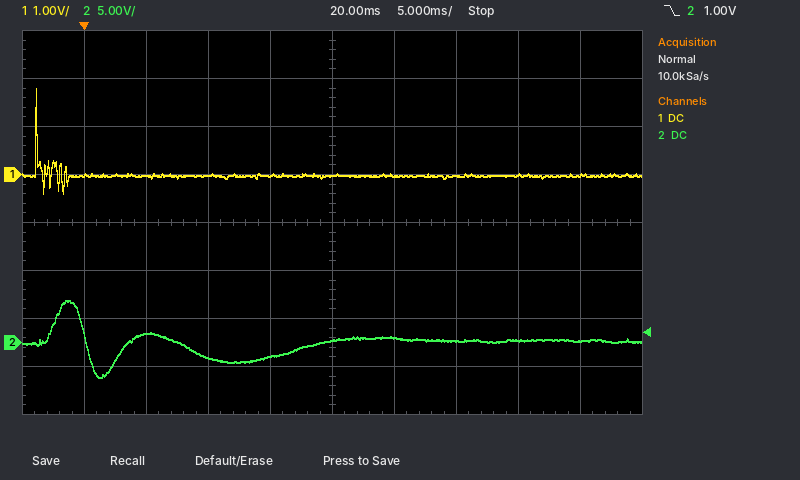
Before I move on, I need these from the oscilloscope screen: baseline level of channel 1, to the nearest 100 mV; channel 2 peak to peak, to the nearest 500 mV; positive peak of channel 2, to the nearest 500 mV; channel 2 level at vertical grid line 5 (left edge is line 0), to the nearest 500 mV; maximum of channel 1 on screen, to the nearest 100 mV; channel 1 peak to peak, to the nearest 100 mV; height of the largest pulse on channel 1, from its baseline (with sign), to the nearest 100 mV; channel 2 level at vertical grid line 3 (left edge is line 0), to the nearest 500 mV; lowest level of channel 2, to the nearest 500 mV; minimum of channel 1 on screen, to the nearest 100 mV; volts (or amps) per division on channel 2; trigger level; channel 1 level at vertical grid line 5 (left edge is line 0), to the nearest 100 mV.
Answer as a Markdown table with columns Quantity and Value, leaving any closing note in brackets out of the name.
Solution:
| Quantity | Value |
|---|---|
| baseline level of channel 1, to the nearest 100 mV | 0.0 V |
| channel 2 peak to peak, to the nearest 500 mV | 8.0 V |
| positive peak of channel 2, to the nearest 500 mV | 4.5 V |
| channel 2 level at vertical grid line 5 (left edge is line 0), to the nearest 500 mV | 0.0 V |
| maximum of channel 1 on screen, to the nearest 100 mV | 1.8 V |
| channel 1 peak to peak, to the nearest 100 mV | 2.2 V |
| height of the largest pulse on channel 1, from its baseline (with sign), to the nearest 100 mV | +1.8 V |
| channel 2 level at vertical grid line 3 (left edge is line 0), to the nearest 500 mV | -1.5 V |
| lowest level of channel 2, to the nearest 500 mV | -3.5 V |
| minimum of channel 1 on screen, to the nearest 100 mV | -400 mV |
| volts (or amps) per division on channel 2 | 5 V |
| trigger level | 1.00 V |
| channel 1 level at vertical grid line 5 (left edge is line 0), to the nearest 100 mV | 0.0 V |
